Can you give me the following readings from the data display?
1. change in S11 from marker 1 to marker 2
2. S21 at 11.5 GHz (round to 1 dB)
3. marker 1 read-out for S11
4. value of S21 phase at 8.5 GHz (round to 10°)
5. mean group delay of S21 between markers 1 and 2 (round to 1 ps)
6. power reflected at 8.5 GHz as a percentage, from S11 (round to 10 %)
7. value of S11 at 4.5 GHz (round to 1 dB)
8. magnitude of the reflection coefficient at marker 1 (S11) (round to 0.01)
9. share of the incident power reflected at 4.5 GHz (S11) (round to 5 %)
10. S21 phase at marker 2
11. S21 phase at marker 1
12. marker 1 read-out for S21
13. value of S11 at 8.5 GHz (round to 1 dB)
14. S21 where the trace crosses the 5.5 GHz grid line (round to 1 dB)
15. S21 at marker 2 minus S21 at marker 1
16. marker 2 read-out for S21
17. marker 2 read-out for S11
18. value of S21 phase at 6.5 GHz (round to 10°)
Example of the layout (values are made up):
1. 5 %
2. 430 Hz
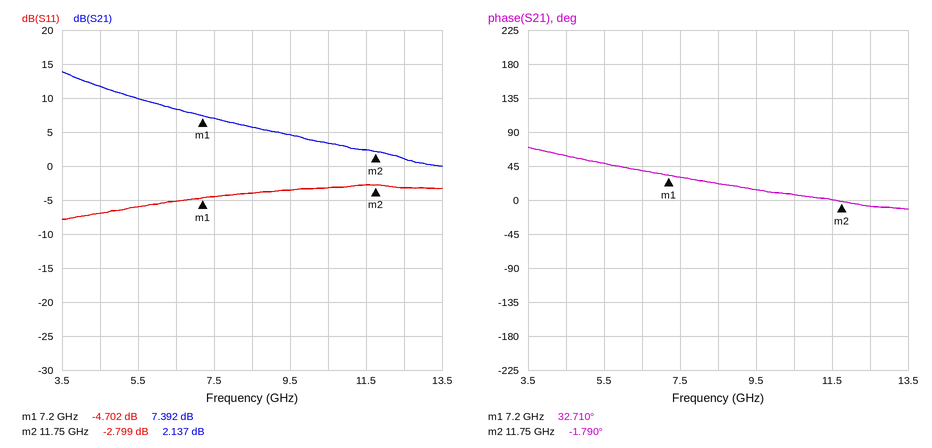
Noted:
1. 1.903 dB
2. 2 dB
3. -4.702 dB
4. 20°
5. 21 ps
6. 40 %
7. -7 dB
8. 0.58
9. 20 %
10. -1.790°
11. 32.710°
12. 7.392 dB
13. -4 dB
14. 10 dB
15. -5.255 dB
16. 2.137 dB
17. -2.799 dB
18. 40°
